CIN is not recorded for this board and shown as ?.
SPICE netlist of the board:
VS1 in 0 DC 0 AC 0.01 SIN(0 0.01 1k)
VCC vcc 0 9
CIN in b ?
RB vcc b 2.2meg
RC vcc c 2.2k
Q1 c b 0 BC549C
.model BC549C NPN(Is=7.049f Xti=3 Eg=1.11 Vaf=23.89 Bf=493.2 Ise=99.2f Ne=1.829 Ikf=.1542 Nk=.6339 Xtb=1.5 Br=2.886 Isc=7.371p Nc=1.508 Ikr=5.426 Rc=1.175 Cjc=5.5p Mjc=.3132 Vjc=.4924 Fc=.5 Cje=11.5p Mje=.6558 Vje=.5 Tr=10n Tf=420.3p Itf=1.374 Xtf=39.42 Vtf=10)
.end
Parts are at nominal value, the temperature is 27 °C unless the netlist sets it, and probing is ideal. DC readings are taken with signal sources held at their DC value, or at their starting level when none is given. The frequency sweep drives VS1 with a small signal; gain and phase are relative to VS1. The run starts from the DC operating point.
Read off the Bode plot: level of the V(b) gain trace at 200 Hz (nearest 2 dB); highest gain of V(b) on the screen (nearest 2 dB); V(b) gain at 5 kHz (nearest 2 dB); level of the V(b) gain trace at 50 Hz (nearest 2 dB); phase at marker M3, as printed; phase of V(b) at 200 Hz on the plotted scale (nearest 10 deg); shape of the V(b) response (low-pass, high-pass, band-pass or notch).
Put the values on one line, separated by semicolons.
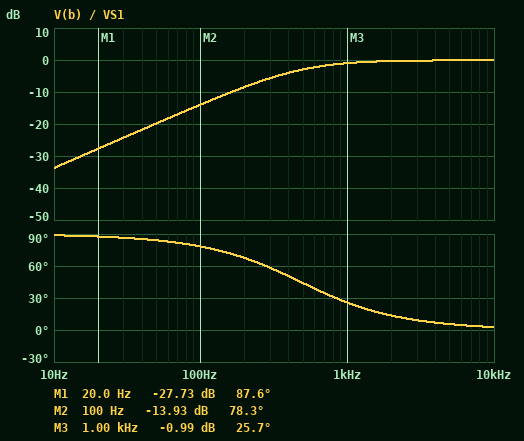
-8 dB; 0 dB; 0 dB; -20 dB; 25.7 deg; 70 deg; high-pass
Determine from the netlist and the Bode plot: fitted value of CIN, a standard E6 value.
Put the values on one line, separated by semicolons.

47 nF
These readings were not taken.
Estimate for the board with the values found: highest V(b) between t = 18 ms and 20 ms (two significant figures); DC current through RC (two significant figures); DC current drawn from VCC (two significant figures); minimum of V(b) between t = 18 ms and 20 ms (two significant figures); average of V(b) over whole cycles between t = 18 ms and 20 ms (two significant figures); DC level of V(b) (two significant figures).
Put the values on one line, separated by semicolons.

690 mV; 2.0 mA; 2.0 mA; 670 mV; 680 mV; 680 mV
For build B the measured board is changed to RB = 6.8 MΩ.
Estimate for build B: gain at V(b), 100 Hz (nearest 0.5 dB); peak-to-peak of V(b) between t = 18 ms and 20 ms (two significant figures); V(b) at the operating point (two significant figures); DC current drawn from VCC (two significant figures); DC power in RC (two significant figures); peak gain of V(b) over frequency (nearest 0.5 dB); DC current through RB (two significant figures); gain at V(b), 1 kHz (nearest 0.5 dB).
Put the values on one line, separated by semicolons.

-5.5 dB; 20 mV; 650 mV; 720 µA; 1.1 mW; 0 dB; 1.2 µA; 0 dB
